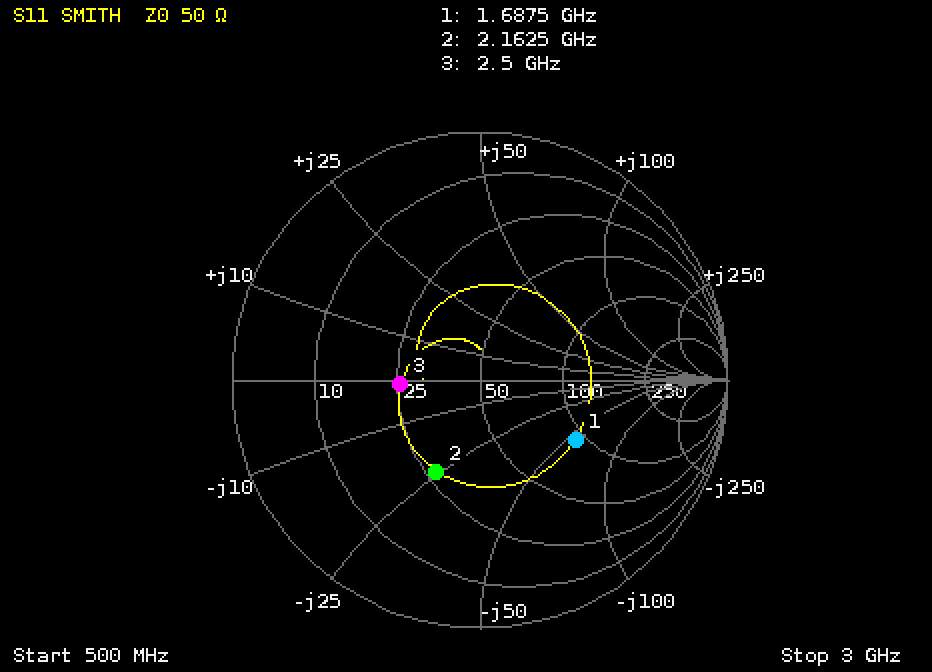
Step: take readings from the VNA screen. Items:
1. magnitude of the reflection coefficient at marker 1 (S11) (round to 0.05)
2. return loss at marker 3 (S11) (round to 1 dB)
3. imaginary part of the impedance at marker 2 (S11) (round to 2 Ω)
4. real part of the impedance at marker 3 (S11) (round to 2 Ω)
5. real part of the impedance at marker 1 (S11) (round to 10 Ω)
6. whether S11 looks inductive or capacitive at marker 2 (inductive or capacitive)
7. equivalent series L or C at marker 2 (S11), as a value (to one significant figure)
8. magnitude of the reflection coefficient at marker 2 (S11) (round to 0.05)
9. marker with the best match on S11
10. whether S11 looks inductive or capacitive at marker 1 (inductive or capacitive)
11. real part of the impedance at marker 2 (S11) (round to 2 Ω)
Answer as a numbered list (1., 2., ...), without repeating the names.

1. 0.45
2. 10 dB
3. -24 Ω
4. 26 Ω
5. 90 Ω
6. capacitive
7. 3 pF
8. 0.40
9. marker 3
10. capacitive
11. 28 Ω
